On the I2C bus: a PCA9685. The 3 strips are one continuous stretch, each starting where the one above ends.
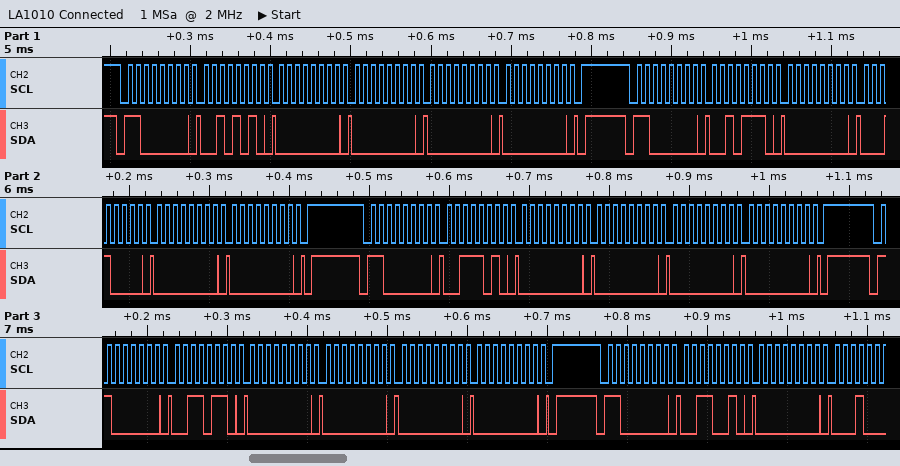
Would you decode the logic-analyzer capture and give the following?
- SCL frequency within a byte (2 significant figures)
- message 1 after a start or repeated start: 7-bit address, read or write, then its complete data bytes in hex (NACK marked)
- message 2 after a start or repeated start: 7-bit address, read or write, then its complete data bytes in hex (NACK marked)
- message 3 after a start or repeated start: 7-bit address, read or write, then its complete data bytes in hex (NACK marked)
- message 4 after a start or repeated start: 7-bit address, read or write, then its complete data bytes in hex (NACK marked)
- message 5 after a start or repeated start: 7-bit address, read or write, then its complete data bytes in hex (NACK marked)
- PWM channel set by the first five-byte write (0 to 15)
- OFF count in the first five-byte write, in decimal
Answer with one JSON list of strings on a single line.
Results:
["100 kHz", "0x60 write: 2A 00 00 00 00", "0x60 write: 2E 00 10 00 00", "0x60 write: 3A 00 00 00 00", "0x60 write: 36 00 00 00 00", "0x60 write: 32 00", "9", "0"]
